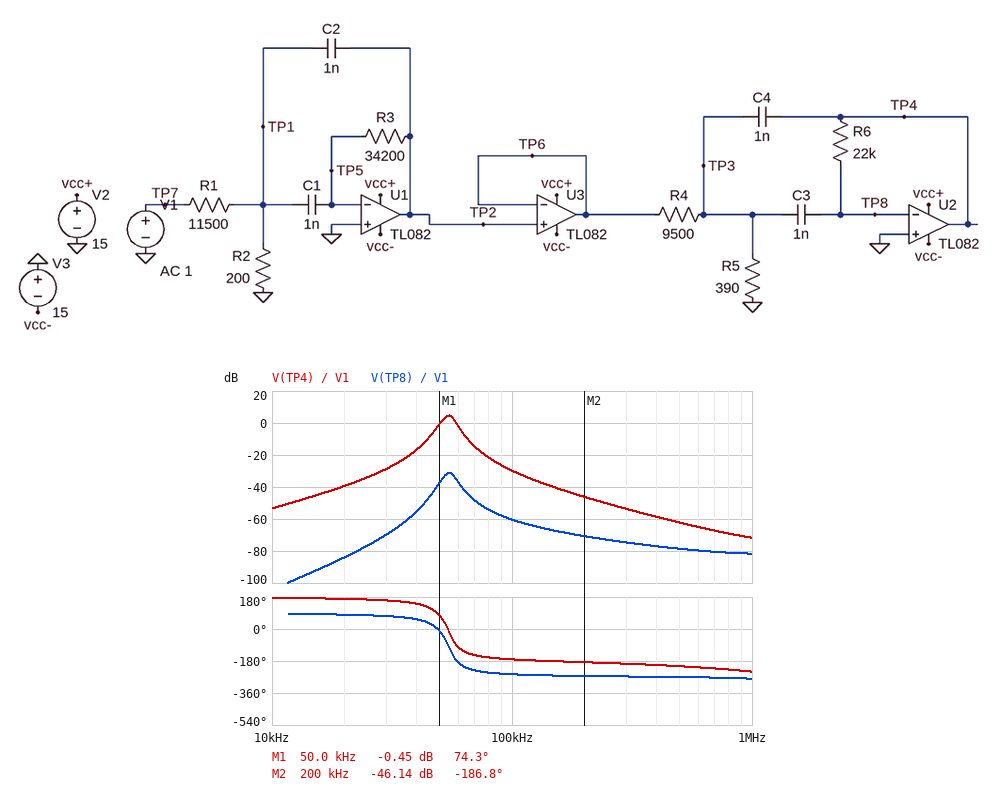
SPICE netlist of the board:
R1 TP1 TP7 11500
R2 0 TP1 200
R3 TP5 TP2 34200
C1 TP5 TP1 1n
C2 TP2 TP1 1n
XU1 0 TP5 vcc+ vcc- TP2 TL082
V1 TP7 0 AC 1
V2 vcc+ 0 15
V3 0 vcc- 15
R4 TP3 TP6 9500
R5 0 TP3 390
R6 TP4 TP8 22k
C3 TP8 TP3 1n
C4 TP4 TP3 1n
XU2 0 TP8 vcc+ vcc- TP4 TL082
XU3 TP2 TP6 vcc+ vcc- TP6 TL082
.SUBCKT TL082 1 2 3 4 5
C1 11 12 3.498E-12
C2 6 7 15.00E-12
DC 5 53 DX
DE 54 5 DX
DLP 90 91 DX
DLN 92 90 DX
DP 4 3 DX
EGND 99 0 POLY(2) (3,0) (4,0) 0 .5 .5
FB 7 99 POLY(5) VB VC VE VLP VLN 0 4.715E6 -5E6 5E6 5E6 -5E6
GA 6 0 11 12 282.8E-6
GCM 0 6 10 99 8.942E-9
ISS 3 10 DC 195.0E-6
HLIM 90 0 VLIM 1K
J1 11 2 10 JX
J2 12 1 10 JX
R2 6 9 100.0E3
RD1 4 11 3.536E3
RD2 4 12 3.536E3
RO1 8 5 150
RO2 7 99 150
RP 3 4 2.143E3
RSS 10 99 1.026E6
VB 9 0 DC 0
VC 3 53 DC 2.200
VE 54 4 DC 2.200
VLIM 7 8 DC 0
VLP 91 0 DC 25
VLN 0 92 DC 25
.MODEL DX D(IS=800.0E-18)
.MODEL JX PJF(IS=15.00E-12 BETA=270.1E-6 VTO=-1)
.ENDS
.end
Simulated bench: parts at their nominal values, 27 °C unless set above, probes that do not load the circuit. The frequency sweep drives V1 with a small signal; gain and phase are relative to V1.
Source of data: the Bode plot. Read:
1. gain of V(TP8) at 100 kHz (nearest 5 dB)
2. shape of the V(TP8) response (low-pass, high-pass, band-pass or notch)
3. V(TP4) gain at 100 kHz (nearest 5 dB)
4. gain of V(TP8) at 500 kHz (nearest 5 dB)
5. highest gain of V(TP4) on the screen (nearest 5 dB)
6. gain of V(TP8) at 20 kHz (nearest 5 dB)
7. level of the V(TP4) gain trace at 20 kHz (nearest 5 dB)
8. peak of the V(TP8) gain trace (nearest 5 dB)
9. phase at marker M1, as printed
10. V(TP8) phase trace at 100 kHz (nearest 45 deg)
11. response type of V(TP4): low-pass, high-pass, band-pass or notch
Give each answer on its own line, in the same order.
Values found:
-60 dB
band-pass
-30 dB
-80 dB
5 dB
-85 dB
-40 dB
-30 dB
74.3 deg
-270 deg
band-pass
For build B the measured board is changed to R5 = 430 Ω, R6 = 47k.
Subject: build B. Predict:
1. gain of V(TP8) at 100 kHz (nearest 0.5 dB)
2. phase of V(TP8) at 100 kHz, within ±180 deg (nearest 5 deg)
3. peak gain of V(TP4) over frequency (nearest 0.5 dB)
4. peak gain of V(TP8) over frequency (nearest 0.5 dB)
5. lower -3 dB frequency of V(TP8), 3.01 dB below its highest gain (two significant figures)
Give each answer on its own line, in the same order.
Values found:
-62.0 dB
100 deg
-3.0 dB
-39.0 dB
51 kHz
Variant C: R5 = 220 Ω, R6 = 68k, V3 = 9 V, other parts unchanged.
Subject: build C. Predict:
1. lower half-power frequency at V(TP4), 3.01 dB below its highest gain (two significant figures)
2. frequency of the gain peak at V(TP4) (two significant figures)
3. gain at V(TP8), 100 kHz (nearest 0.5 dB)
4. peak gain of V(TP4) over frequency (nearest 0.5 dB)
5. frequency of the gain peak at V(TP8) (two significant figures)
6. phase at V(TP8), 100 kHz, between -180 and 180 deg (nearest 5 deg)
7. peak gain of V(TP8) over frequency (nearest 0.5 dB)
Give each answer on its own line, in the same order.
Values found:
36 kHz
38 kHz
-62.5 dB
0 dB
55 kHz
100 deg
-38.5 dB
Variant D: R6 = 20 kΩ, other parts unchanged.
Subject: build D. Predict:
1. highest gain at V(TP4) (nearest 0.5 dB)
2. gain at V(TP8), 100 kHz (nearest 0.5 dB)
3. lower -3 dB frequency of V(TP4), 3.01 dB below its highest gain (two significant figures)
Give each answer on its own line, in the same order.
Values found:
4.5 dB
-60.0 dB
52 kHz
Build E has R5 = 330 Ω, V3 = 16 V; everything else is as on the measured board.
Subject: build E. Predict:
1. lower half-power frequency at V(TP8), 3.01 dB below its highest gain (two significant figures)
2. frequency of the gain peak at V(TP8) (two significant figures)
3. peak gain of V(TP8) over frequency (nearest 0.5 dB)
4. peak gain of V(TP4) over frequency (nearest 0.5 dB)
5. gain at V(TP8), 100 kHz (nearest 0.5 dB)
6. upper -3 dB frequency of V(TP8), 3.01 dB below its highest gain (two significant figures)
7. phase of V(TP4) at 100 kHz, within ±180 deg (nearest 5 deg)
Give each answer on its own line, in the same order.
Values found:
53 kHz
56 kHz
-30.5 dB
5.5 dB
-60.0 dB
59 kHz
-170 deg
